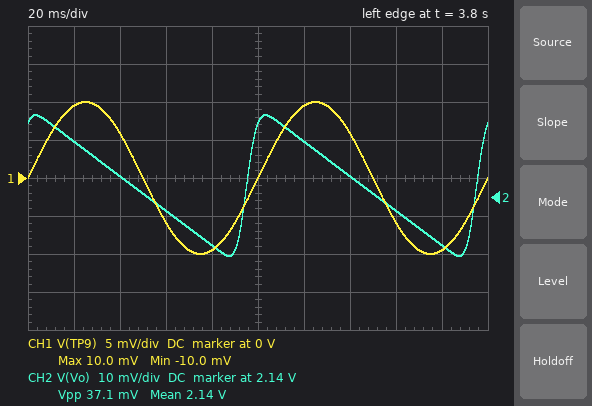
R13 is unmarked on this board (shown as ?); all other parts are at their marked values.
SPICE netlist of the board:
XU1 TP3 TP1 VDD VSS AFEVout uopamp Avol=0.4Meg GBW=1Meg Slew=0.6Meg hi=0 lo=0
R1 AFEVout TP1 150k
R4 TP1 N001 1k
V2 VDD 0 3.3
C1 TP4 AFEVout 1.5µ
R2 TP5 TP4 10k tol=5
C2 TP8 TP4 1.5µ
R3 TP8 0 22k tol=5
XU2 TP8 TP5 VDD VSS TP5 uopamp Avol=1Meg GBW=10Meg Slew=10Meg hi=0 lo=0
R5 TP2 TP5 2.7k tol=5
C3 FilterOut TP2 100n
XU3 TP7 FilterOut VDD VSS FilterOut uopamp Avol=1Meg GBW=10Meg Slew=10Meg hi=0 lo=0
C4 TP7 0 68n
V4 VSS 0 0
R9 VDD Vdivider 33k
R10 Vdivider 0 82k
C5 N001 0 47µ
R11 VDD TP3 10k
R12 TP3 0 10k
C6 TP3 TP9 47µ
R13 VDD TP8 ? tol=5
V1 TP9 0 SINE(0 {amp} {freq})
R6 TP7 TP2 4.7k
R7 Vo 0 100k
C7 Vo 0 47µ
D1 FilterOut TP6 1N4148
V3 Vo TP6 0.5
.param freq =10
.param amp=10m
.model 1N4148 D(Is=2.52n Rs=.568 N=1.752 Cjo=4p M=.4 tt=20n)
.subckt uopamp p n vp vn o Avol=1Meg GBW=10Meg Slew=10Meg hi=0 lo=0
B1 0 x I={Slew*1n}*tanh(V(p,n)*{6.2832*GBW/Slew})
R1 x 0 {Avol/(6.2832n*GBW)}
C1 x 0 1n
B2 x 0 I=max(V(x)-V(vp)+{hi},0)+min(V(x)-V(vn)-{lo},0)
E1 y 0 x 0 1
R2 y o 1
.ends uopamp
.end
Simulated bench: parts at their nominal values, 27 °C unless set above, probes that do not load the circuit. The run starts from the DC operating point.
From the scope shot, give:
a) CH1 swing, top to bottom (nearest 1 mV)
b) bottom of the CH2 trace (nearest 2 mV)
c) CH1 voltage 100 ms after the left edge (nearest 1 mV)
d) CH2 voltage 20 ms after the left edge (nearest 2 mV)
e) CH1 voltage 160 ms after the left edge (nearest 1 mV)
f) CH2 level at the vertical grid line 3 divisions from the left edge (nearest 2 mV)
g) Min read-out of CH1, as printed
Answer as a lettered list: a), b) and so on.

a) 20 mV
b) 2.124 V
c) 0 V
d) 2.154 V
e) -6 mV
f) 2.136 V
g) -10.0 mV
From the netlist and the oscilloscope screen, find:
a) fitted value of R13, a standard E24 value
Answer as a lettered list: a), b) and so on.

a) 36 kΩ
